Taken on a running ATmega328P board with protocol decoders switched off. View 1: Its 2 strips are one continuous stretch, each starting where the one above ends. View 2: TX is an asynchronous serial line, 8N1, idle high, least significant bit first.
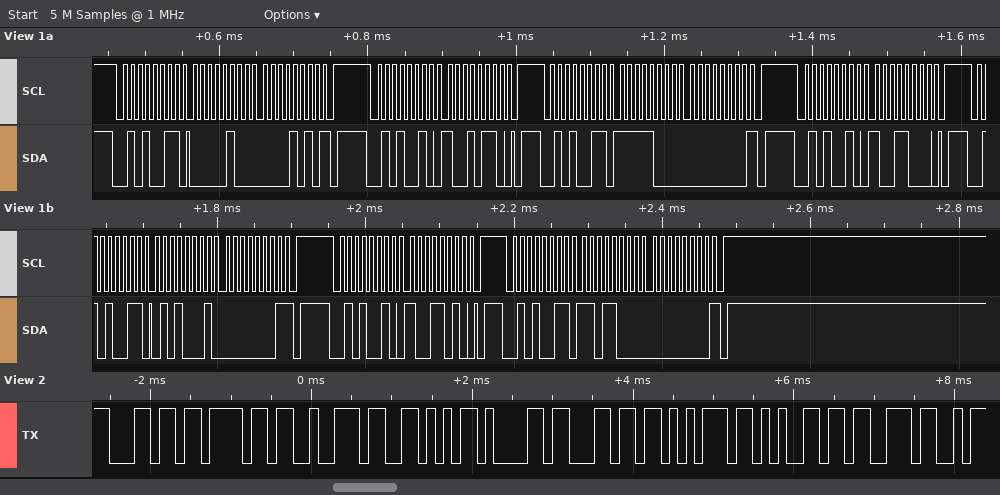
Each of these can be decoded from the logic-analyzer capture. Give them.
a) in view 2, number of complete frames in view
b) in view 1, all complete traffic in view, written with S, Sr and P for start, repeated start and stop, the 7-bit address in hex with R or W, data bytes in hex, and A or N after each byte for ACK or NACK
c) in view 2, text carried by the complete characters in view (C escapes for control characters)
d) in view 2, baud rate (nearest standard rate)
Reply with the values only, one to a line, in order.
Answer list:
9
S 29R A 04 A 0A N P S 29W A 96 A P S 29R A F8 A 00 N P S 29W A 98 A P S 29R A 51 A 01 N P S 29W A 9A A P S 29R A D8 A 00 N P
"lorValues"
9600 baud
